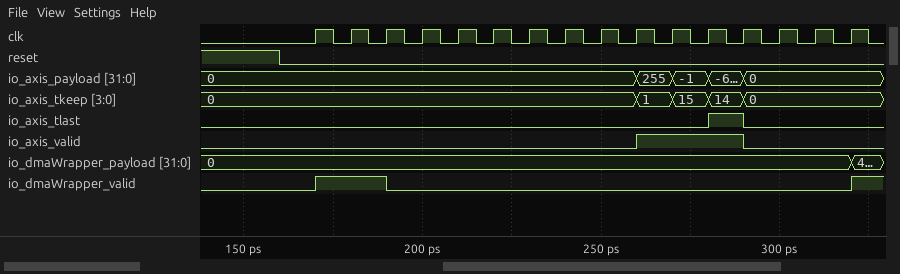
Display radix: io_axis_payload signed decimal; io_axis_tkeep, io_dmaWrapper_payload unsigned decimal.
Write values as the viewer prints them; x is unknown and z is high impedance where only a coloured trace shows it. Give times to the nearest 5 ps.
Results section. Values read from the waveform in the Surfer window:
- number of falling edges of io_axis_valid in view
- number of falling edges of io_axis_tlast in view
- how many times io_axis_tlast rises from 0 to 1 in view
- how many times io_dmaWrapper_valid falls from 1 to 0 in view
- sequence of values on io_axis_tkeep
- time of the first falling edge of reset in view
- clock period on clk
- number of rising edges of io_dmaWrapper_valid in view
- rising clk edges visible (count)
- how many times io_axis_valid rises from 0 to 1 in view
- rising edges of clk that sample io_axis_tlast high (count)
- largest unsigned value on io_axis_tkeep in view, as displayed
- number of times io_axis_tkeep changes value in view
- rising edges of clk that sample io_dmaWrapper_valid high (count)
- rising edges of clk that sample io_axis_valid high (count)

1
1
1
1
0, 1, 15, 14, 0
160 ps
10 ps
2
16
1
1
15
4
2
3
